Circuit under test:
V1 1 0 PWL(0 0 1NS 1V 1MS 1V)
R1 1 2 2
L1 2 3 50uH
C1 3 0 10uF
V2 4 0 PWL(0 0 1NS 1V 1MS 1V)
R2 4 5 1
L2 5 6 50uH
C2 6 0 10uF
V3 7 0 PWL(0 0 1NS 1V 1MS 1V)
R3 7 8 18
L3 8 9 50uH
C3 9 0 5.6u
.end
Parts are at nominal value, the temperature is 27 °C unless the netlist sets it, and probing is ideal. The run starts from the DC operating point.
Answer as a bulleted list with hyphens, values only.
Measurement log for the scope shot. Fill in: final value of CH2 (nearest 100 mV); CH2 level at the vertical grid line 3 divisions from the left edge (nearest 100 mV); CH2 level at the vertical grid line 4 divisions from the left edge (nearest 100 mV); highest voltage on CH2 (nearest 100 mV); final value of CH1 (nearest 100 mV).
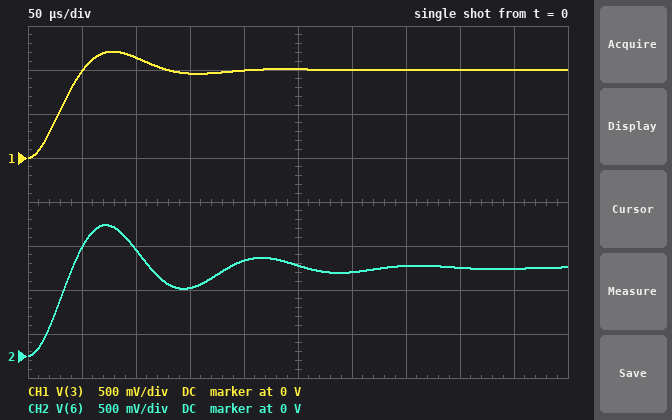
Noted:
- 1.0 V
- 800 mV
- 1.1 V
- 1.5 V
- 1.0 V
